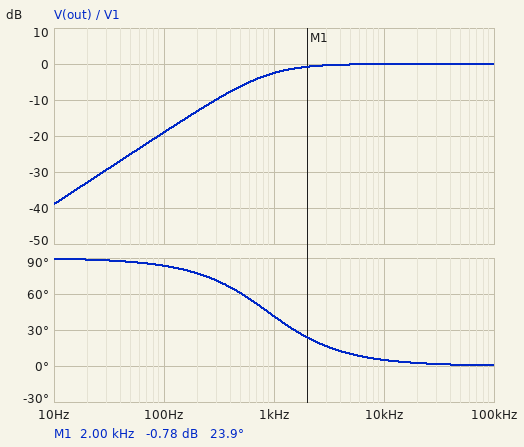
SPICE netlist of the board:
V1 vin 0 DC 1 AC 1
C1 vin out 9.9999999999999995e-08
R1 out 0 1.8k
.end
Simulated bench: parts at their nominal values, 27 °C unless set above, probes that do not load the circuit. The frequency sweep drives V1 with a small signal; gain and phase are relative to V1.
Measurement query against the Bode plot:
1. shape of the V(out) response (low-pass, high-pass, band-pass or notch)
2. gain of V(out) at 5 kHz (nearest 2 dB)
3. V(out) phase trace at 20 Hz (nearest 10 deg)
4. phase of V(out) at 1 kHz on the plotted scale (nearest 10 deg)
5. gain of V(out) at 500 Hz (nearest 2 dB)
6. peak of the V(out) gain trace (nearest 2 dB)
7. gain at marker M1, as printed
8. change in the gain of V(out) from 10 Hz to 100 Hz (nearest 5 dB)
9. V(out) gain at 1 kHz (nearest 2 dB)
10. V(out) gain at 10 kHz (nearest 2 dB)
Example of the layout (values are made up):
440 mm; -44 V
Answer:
high-pass; 0 dB; 90 deg; 40 deg; -6 dB; 0 dB; -0.78 dB; 20 dB; -2 dB; 0 dB
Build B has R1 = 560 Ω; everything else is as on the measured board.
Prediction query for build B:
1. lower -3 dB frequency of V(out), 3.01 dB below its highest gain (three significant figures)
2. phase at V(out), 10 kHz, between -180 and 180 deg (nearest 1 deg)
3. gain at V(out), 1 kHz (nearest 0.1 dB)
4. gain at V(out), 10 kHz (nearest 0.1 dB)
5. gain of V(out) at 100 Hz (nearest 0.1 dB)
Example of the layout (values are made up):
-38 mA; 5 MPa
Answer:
2.84 kHz; 16 deg; -9.6 dB; -0.3 dB; -29.1 dB
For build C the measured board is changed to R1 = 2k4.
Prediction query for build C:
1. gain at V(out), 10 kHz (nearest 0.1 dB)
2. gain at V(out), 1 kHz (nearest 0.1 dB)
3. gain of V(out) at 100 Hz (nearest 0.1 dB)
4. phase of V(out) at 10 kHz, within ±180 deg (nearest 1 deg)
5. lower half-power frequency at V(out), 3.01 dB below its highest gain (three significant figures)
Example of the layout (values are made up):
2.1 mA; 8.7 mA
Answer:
0 dB; -1.6 dB; -16.5 dB; 4 deg; 663 Hz
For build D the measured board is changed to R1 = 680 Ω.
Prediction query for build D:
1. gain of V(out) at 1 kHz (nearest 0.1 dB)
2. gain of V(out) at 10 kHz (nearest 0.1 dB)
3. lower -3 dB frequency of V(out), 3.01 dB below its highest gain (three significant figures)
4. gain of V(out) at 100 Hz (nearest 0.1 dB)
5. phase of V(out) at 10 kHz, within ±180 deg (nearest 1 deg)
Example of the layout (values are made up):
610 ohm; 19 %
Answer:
-8.1 dB; -0.2 dB; 2.34 kHz; -27.4 dB; 13 deg
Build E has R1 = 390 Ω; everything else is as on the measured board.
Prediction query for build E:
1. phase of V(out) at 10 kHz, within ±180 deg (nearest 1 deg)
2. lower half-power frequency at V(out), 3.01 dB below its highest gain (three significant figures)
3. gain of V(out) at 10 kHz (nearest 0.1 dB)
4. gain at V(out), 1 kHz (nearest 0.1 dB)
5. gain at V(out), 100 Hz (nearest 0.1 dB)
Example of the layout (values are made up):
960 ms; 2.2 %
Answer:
22 deg; 4.08 kHz; -0.7 dB; -12.5 dB; -32.2 dB
